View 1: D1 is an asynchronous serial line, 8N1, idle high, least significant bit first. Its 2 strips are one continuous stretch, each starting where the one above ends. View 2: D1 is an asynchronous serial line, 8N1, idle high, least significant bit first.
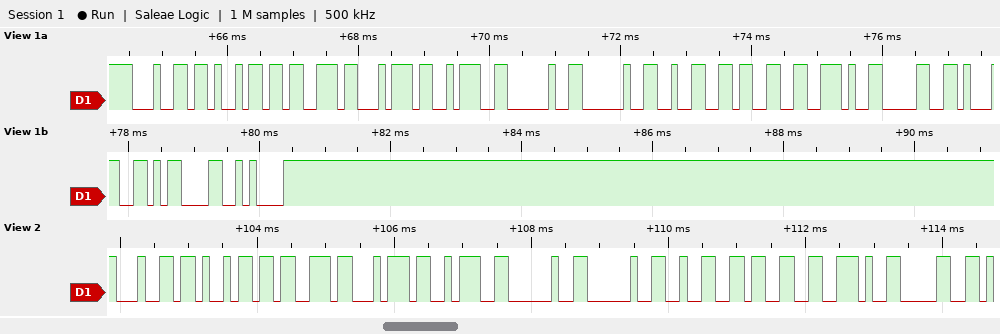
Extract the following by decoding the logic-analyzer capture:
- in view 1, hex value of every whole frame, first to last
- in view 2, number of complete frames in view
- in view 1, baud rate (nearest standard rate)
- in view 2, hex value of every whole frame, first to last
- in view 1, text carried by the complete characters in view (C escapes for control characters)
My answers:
64 69 73 74 3A 20 20 32 33 2E 30 31 0D 0A
11
9600 baud
64 69 73 74 3A 20 20 32 33 2E 30
"dist:  23.01\r\n"
